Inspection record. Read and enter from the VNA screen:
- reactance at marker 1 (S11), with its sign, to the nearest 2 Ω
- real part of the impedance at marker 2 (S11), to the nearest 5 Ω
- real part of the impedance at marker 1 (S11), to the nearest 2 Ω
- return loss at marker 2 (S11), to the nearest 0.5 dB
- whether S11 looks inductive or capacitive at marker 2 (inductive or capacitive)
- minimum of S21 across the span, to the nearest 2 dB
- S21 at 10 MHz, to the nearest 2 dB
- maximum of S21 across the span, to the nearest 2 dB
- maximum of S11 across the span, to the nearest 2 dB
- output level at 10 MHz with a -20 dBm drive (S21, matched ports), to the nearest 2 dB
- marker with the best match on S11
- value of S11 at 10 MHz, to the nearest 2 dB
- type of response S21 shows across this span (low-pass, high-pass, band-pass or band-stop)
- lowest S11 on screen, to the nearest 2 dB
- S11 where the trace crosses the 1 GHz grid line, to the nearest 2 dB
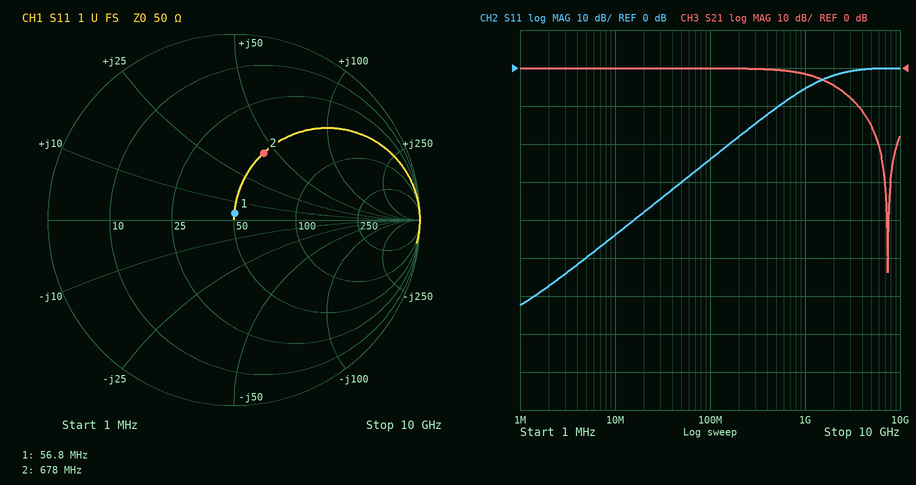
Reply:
+4 Ω
50 Ω
50 Ω
8.0 dB
inductive
-54 dB
0 dB
0 dB
0 dB
-20 dBm
marker 1
-44 dB
low-pass
-62 dB
-6 dB
